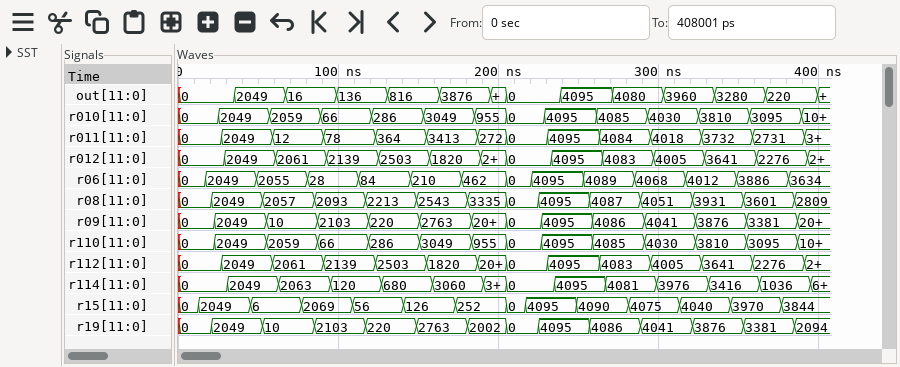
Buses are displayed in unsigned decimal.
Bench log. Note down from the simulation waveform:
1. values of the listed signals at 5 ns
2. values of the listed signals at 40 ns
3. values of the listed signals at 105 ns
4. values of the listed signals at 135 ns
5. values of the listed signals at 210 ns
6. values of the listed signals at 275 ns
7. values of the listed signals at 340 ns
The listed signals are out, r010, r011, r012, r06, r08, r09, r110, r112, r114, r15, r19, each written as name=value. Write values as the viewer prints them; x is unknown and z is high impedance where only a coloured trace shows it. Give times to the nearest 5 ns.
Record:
out=0, r010=0, r011=0, r012=0, r06=0, r08=0, r09=0, r110=0, r112=0, r114=0, r15=0, r19=0
out=2049, r010=2049, r011=2049, r012=2049, r06=2049, r08=2049, r09=2049, r110=2049, r112=2049, r114=2049, r15=2049, r19=2049
out=136, r010=66, r011=78, r012=2139, r06=28, r08=2093, r09=2103, r110=66, r112=2139, r114=120, r15=2069, r19=2103
out=816, r010=286, r011=364, r012=2503, r06=84, r08=2213, r09=220, r110=286, r112=2503, r114=680, r15=56, r19=220
out=0, r010=0, r011=0, r012=0, r06=0, r08=0, r09=0, r110=0, r112=0, r114=0, r15=0, r19=0
out=4080, r010=4085, r011=4084, r012=4083, r06=4089, r08=4087, r09=4086, r110=4085, r112=4083, r114=4081, r15=4090, r19=4086
out=3280, r010=3810, r011=3732, r012=3641, r06=4012, r08=3931, r09=3876, r110=3810, r112=3641, r114=3416, r15=4040, r19=3876
